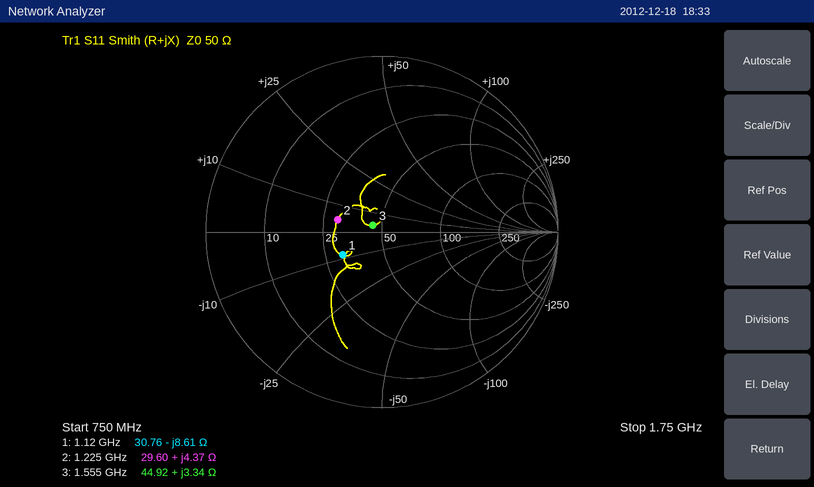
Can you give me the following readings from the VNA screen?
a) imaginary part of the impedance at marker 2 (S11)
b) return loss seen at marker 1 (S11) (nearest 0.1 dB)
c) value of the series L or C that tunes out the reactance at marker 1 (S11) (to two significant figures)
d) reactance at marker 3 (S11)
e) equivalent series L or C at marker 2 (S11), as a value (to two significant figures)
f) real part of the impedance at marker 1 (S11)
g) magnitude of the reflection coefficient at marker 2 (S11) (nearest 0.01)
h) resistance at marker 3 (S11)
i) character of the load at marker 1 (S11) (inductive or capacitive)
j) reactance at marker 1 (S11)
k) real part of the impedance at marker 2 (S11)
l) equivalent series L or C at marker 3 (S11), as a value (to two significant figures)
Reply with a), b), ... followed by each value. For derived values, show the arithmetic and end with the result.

a) +4.37 Ω
b) 11.7 dB
c) L = 8.61 Ω/(2π × 1.12 GHz) ≈ 1.2 nH
d) +3.34 Ω
e) L = 4.37 Ω/(2π × 1.225 GHz) ≈ 568 pH, so 570 pH to two significant figures
f) 30.76 Ω
g) 0.26
h) 44.92 Ω
i) capacitive
j) -8.61 Ω
k) 29.60 Ω
l) L = 3.34 Ω/(2π × 1.555 GHz) ≈ 342 pH, so 340 pH to two significant figures
